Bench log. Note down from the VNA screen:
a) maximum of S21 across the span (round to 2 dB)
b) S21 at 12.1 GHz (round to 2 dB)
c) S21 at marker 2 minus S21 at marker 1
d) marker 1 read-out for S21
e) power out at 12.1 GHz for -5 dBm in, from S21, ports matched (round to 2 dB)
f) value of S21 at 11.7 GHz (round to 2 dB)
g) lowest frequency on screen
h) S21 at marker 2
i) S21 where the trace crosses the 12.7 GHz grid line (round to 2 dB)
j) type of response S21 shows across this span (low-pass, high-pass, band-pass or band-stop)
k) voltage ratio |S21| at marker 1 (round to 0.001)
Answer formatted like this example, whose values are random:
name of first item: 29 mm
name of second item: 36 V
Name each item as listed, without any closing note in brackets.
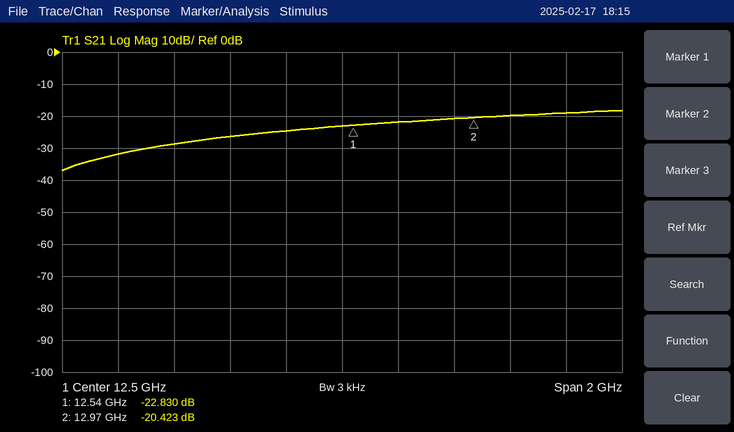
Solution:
maximum of S21 across the span: -18 dB
S21 at 12.1 GHz: -26 dB
S21 at marker 2 minus S21 at marker 1: 2.407 dB
marker 1 read-out for S21: -22.830 dB
power out at 12.1 GHz for -5 dBm in, from S21, ports matched: -32 dBm
value of S21 at 11.7 GHz: -32 dB
lowest frequency on screen: 11.5 GHz
S21 at marker 2: -20.423 dB
S21 where the trace crosses the 12.7 GHz grid line: -22 dB
type of response S21 shows across this span: high-pass
voltage ratio |S21| at marker 1: 0.072
